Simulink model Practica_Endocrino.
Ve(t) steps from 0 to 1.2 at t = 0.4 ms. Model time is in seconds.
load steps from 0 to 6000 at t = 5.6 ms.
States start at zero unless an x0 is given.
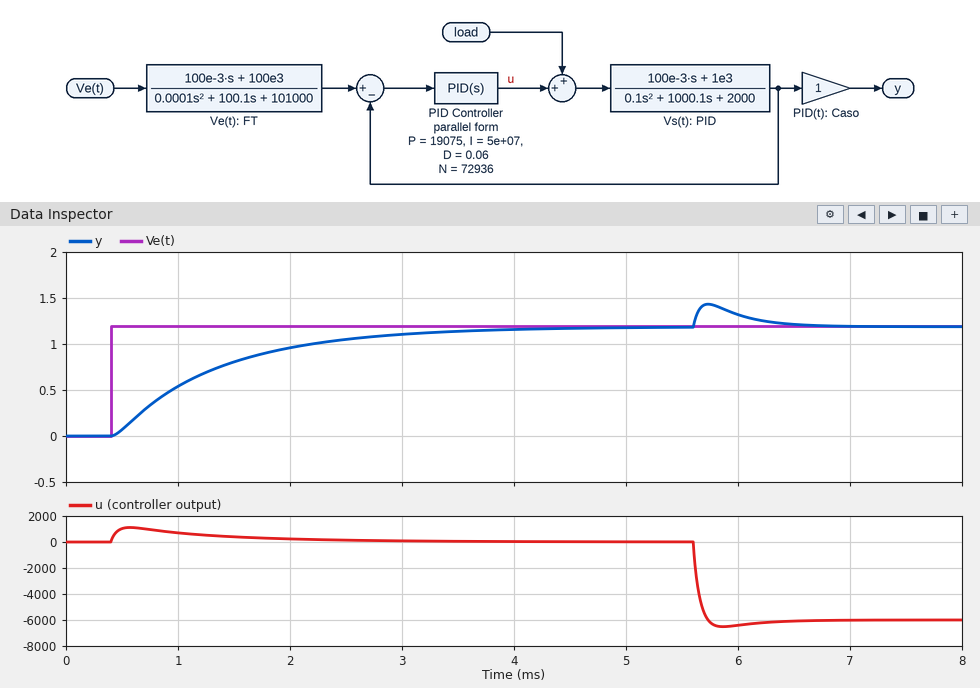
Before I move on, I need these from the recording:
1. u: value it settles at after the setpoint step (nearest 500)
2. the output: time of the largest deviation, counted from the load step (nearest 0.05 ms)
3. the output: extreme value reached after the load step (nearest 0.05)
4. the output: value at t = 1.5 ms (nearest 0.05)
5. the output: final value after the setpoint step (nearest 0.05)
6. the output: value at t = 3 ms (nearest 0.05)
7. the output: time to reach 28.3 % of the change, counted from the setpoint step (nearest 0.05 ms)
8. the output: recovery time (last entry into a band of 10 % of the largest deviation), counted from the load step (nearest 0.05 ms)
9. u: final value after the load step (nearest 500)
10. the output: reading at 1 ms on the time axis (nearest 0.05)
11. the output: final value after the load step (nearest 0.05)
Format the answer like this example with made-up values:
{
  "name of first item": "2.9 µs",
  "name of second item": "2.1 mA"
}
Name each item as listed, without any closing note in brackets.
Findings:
{
  "u: value it settles at after the setpoint step": "0",
  "the output: time of the largest deviation, counted from the load step": "0.15 ms",
  "the output: extreme value reached after the load step": "1.45",
  "the output: value at t = 1.5 ms": "0.80",
  "the output: final value after the setpoint step": "1.20",
  "the output: value at t = 3 ms": "1.10",
  "the output: time to reach 28.3 % of the change, counted from the setpoint step": "0.35 ms",
  "the output: recovery time (last entry into a band of 10 % of the largest deviation), counted from the load step": "0.90 ms",
  "u: final value after the load step": "-6000",
  "the output: reading at 1 ms on the time axis": "0.55",
  "the output: final value after the load step": "1.20"
}
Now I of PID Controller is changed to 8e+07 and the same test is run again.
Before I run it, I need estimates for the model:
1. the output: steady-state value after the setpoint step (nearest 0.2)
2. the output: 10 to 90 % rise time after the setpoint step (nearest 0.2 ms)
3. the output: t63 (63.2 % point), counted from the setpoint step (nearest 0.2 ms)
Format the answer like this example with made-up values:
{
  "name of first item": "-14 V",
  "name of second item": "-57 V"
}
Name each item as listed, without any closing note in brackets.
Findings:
{
  "the output: steady-state value after the setpoint step": "1.2",
  "the output: 10 to 90 % rise time after the setpoint step": "2.2 ms",
  "the output: t63 (63.2 % point), counted from the setpoint step": "1.0 ms"
}
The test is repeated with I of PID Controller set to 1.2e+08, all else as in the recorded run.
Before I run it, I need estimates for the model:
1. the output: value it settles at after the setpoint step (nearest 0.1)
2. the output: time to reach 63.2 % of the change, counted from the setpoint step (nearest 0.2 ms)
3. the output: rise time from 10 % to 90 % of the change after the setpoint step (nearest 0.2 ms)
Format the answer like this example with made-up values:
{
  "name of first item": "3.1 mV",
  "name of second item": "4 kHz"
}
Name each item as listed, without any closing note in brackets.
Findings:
{
  "the output: value it settles at after the setpoint step": "1.2",
  "the output: time to reach 63.2 % of the change, counted from the setpoint step": "1.0 ms",
  "the output: rise time from 10 % to 90 % of the change after the setpoint step": "2.2 ms"
}
